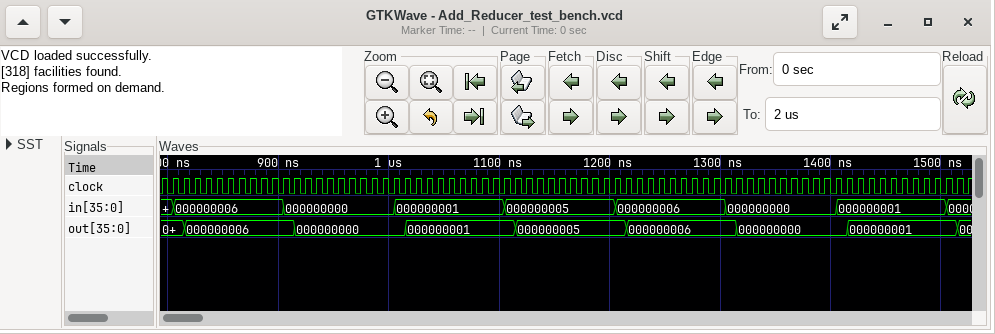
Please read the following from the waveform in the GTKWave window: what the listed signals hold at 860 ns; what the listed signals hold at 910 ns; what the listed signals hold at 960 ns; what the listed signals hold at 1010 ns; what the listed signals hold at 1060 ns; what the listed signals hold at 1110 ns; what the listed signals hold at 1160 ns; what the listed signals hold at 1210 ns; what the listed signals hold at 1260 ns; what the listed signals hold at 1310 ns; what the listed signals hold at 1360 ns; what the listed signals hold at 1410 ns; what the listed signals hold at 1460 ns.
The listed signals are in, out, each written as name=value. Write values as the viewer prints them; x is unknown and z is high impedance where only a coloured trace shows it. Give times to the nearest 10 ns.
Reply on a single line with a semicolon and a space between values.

in=000000006, out=000000006; in=000000000, out=000000006; in=000000000, out=000000000; in=000000001, out=000000000; in=000000001, out=000000001; in=000000005, out=000000001; in=000000005, out=000000005; in=000000006, out=000000005; in=000000006, out=000000006; in=000000000, out=000000006; in=000000000, out=000000000; in=000000001, out=000000000; in=000000001, out=000000001
